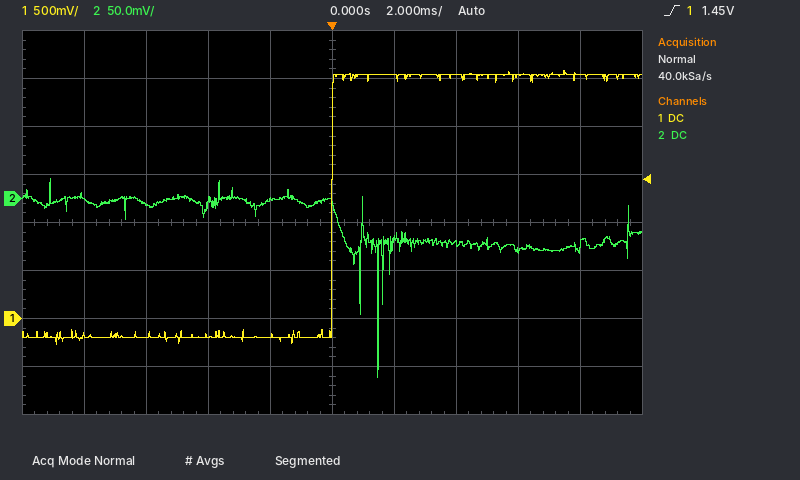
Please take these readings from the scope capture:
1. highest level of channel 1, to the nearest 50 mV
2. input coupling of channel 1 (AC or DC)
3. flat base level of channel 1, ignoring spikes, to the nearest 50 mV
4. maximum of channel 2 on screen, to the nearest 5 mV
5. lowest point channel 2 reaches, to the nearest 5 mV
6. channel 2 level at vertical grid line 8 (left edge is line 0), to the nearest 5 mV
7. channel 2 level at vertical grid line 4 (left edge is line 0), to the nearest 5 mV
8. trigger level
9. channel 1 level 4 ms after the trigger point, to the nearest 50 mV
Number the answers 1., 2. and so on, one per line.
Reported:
1. 2.60 V
2. DC
3. -200 mV
4. 20 mV
5. -185 mV
6. -55 mV
7. 0 mV
8. 1.45 V
9. 2.55 V
